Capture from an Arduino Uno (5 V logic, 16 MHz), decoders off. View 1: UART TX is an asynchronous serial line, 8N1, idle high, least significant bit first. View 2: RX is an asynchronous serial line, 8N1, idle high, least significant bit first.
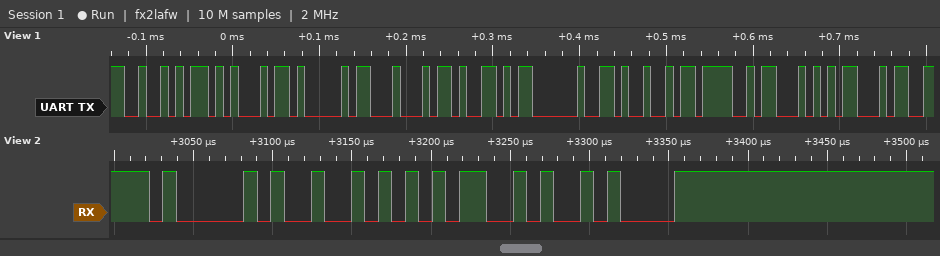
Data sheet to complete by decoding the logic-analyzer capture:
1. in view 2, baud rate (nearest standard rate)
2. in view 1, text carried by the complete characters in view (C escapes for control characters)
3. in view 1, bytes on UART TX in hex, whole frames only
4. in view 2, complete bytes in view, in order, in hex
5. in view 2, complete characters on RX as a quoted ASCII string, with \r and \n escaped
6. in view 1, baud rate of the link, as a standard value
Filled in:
115200 baud
"READY IOT4"
52 45 41 44 59 20 49 4F 54 34
41 52 4D 0A
"ARM\n"
115200 baud
